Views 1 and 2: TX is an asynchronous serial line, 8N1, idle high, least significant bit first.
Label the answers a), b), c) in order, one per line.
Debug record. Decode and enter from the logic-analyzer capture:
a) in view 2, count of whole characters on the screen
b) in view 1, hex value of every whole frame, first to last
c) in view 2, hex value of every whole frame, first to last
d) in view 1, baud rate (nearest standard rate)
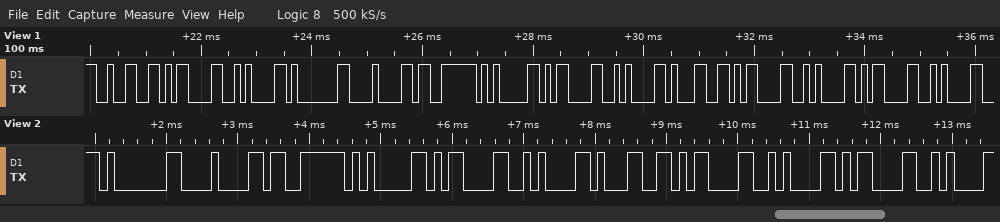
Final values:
a) 11
b) 32 0D 0A 01 08 F3 05 0D 0A 31 0D 0A 0D 0A
c) 01 08 F3 05 0D 0A 31 0D 0A 0D 0A
d) 9600 baud
